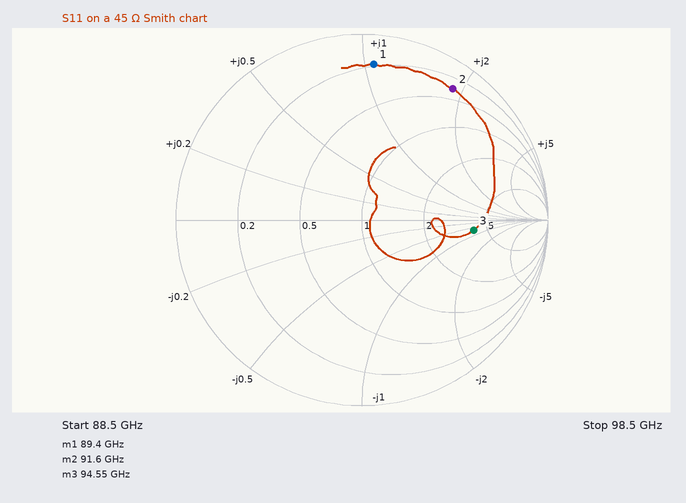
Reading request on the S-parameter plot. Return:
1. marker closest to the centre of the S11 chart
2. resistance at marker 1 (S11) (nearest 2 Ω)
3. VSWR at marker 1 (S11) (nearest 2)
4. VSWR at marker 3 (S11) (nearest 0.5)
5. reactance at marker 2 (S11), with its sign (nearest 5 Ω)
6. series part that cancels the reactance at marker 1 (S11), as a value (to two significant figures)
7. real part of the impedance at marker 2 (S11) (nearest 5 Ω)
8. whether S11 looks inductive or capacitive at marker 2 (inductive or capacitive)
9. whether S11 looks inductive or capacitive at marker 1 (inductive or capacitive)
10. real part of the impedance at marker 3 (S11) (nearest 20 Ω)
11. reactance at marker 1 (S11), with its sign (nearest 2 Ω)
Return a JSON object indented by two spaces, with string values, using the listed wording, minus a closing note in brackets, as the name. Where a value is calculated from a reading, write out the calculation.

{
  "marker closest to the centre of the S11 chart": "marker 3",
  "resistance at marker 1 (S11)": "8 Ω",
  "VSWR at marker 1 (S11)": "12",
  "VSWR at marker 3 (S11)": "4.0",
  "reactance at marker 2 (S11), with its sign": "+85 Ω",
  "series part that cancels the reactance at marker 1 (S11), as a value": "C = 1/(2π × 89.4 GHz × 48 Ω) ≈ 37 fF",
  "real part of the impedance at marker 2 (S11)": "15 Ω",
  "whether S11 looks inductive or capacitive at marker 2": "inductive",
  "whether S11 looks inductive or capacitive at marker 1": "inductive",
  "real part of the impedance at marker 3 (S11)": "180 Ω",
  "reactance at marker 1 (S11), with its sign": "+48 Ω"
}
